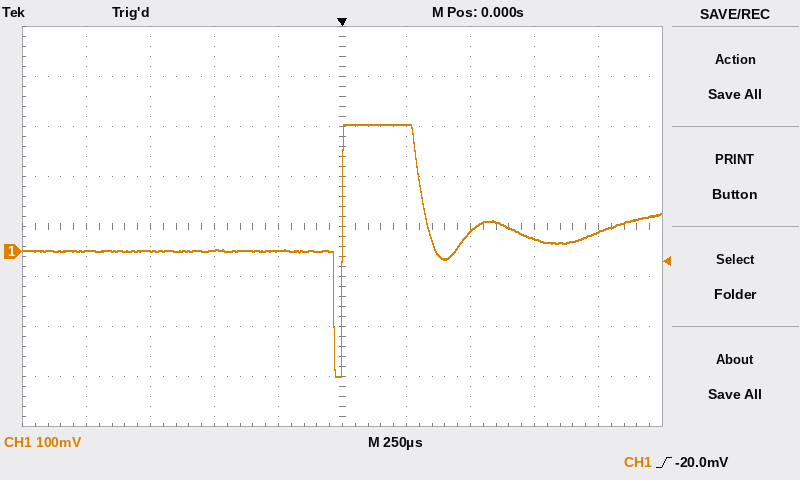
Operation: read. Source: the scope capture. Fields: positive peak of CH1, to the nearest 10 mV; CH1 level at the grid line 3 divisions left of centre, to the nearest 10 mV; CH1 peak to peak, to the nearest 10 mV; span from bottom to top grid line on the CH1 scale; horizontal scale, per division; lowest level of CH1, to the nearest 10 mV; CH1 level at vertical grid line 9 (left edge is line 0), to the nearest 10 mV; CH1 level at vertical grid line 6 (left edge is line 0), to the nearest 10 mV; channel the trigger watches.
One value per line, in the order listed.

250 mV
0 mV
500 mV
800 mV
250 µs
-250 mV
40 mV
250 mV
CH1
